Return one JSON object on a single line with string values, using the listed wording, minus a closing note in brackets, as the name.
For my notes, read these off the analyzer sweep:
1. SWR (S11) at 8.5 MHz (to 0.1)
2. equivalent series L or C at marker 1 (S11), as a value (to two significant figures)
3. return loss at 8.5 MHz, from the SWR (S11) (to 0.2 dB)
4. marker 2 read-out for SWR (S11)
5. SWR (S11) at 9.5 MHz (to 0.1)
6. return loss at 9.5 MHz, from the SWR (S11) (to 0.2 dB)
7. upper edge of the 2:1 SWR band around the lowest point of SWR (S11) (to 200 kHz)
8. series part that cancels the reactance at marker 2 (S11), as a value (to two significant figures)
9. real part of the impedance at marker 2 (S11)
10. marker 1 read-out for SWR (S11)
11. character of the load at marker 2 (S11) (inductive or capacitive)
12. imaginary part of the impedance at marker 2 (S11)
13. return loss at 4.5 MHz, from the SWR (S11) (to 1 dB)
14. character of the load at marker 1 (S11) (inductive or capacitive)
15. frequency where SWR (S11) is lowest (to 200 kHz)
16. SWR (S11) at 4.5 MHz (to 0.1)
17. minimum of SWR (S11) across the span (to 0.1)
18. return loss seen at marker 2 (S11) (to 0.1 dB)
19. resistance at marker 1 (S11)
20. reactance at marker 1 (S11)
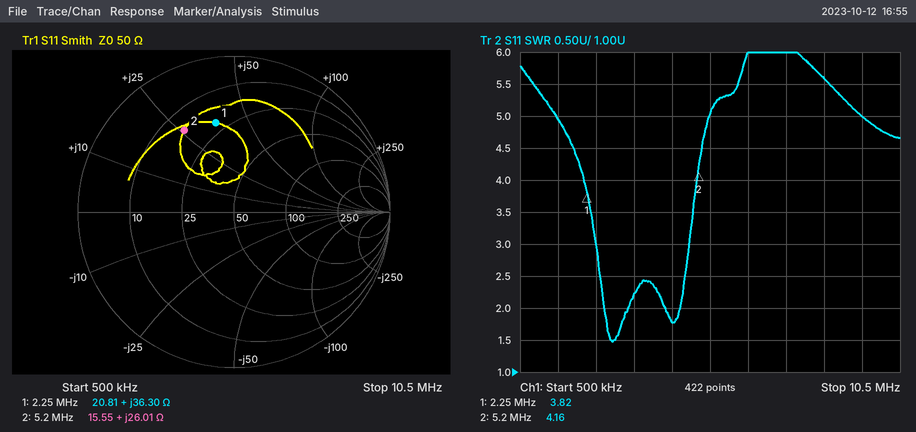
{"SWR (S11) at 8.5 MHz": "5.6", "equivalent series L or C at marker 1 (S11), as a value": "2.6 µH", "return loss at 8.5 MHz, from the SWR (S11)": "3.2 dB", "marker 2 read-out for SWR": "4.16", "SWR (S11) at 9.5 MHz": "5.0", "return loss at 9.5 MHz, from the SWR (S11)": "3.6 dB", "upper edge of the 2:1 SWR band around the lowest point of SWR (S11)": "3.4 MHz", "series part that cancels the reactance at marker 2 (S11), as a value": "1.2 nF", "real part of the impedance at marker 2": "15.55 Ω", "marker 1 read-out for SWR": "3.82", "character of the load at marker 2 (S11)": "inductive", "imaginary part of the impedance at marker 2": "+26.01 Ω", "return loss at 4.5 MHz, from the SWR (S11)": "11 dB", "character of the load at marker 1 (S11)": "inductive", "frequency where SWR (S11) is lowest": "3.0 MHz", "SWR (S11) at 4.5 MHz": "1.8", "minimum of SWR (S11) across the span": "1.5", "return loss seen at marker 2 (S11)": "4.3 dB", "resistance at marker 1": "20.81 Ω", "reactance at marker 1": "+36.30 Ω"}
